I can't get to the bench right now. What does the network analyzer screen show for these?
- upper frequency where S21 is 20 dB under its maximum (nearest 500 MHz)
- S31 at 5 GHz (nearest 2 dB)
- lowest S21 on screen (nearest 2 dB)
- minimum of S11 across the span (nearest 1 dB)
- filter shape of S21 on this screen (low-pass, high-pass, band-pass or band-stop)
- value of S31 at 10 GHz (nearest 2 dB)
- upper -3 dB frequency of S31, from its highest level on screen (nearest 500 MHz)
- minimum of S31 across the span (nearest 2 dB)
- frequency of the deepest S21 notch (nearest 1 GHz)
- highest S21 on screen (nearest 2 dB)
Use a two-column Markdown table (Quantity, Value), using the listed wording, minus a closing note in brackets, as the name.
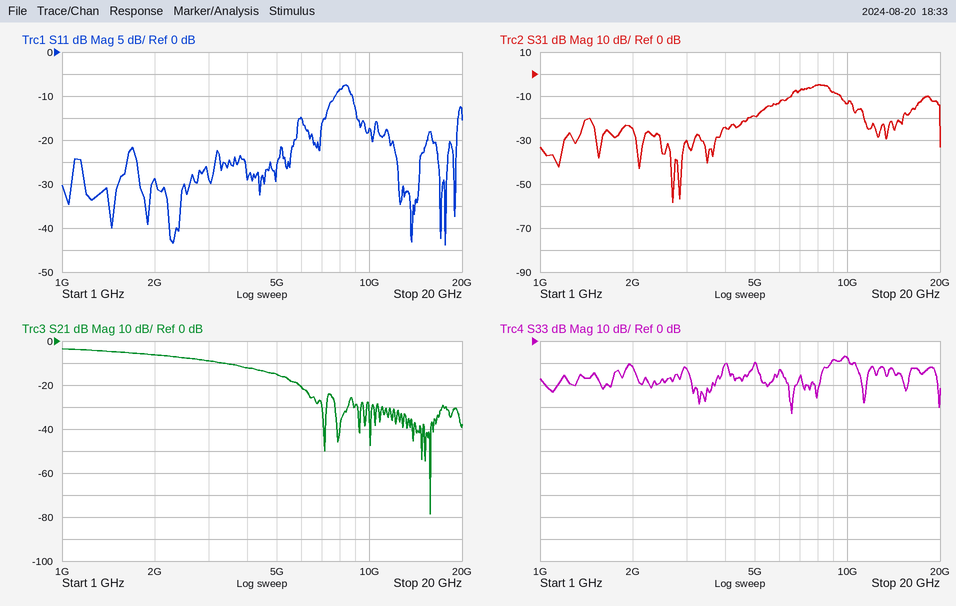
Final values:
| Quantity | Value |
|---|---|
| upper frequency where S21 is 20 dB under its maximum | 6.5 GHz |
| S31 at 5 GHz | -20 dB |
| lowest S21 on screen | -78 dB |
| minimum of S11 across the span | -44 dB |
| filter shape of S21 on this screen | low-pass |
| value of S31 at 10 GHz | -14 dB |
| upper -3 dB frequency of S31, from its highest level on screen | 9.0 GHz |
| minimum of S31 across the span | -58 dB |
| frequency of the deepest S21 notch | 16 GHz |
| highest S21 on screen | -4 dB |
